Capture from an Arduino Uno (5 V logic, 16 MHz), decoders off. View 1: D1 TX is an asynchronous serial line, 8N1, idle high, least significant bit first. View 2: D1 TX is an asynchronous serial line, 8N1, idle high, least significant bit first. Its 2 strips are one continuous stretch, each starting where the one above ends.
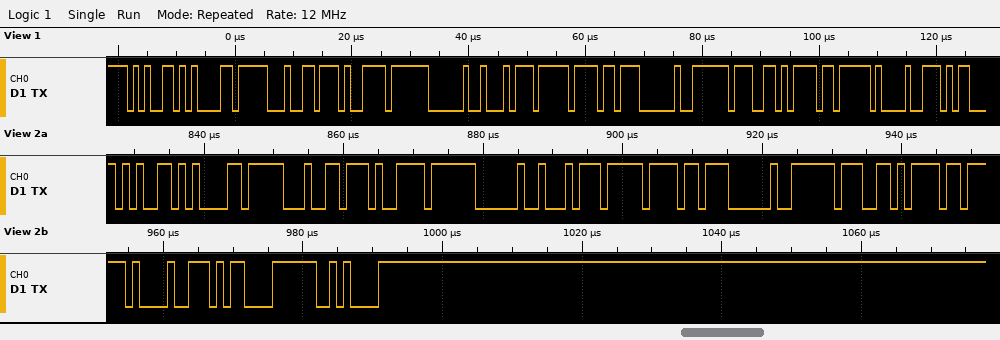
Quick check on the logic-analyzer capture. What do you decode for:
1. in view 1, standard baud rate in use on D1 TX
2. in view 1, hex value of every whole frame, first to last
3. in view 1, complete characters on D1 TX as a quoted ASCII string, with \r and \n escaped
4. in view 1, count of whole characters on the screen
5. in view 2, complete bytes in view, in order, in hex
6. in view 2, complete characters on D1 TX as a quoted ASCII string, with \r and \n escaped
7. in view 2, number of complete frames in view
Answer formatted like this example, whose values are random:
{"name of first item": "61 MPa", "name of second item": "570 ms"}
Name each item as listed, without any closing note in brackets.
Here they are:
{"in view 1, standard baud rate in use on D1 TX": "1000000 baud", "in view 1, hex value of every whole frame, first to last": "0x65 0x61 0x64 0x79 0x20 0x74 0x6F 0x20 0x67 0x6F 0x21", "in view 1, complete characters on D1 TX as a quoted ASCII string, with \\r and \\n escaped": "\"eady to go!\"", "in view 1, count of whole characters on the screen": "11", "in view 2, complete bytes in view, in order, in hex": "65 61 64 79 20 74 6F 20 67 6F 21 0D 0A", "in view 2, complete characters on D1 TX as a quoted ASCII string, with \\r and \\n escaped": "\"eady to go!\\r\\n\"", "in view 2, number of complete frames in view": "13"}
